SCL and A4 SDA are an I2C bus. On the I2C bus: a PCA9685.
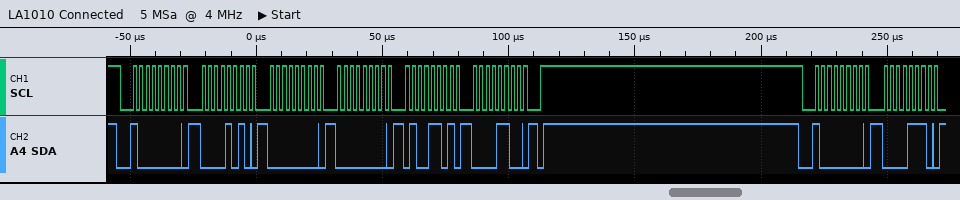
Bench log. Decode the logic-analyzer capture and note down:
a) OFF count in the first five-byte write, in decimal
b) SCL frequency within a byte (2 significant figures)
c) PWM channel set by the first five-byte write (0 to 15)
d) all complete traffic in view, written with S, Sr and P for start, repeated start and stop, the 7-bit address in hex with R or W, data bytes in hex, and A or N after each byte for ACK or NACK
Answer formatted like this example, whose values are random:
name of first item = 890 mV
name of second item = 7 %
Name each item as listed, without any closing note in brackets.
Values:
OFF count in the first five-byte write, in decimal = 3149
SCL frequency within a byte = 400 kHz
PWM channel set by the first five-byte write = 1
all complete traffic in view, written with S, Sr and P for start, repeated start and stop, the 7-bit address in hex with R or W, data bytes in hex, and A or N after each byte for ACK or NACK = S 40W A 0A A 00 A 00 A 4D A 0C A P S 40W A 0E A
